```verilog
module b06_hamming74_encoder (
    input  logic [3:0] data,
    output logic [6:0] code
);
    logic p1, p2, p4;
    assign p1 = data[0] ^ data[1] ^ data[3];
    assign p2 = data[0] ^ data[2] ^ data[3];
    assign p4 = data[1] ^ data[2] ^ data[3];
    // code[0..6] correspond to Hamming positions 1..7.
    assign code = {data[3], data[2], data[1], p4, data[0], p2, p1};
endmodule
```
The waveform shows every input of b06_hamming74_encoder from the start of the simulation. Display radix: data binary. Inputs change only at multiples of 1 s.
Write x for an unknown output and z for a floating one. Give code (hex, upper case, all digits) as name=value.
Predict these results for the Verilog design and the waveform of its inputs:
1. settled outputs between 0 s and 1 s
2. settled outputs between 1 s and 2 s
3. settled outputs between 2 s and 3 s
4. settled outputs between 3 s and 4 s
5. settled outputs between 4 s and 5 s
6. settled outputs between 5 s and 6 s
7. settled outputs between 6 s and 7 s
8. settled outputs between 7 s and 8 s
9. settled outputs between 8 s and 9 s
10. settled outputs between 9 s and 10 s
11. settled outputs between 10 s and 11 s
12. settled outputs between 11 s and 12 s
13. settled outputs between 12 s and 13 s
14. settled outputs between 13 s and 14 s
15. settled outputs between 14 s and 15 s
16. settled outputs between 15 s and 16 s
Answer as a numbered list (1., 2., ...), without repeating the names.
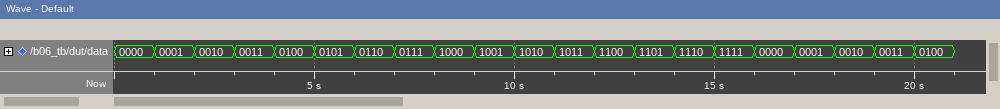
1. code=00
2. code=07
3. code=19
4. code=1E
5. code=2A
6. code=2D
7. code=33
8. code=34
9. code=4B
10. code=4C
11. code=52
12. code=55
13. code=61
14. code=66
15. code=78
16. code=7F
